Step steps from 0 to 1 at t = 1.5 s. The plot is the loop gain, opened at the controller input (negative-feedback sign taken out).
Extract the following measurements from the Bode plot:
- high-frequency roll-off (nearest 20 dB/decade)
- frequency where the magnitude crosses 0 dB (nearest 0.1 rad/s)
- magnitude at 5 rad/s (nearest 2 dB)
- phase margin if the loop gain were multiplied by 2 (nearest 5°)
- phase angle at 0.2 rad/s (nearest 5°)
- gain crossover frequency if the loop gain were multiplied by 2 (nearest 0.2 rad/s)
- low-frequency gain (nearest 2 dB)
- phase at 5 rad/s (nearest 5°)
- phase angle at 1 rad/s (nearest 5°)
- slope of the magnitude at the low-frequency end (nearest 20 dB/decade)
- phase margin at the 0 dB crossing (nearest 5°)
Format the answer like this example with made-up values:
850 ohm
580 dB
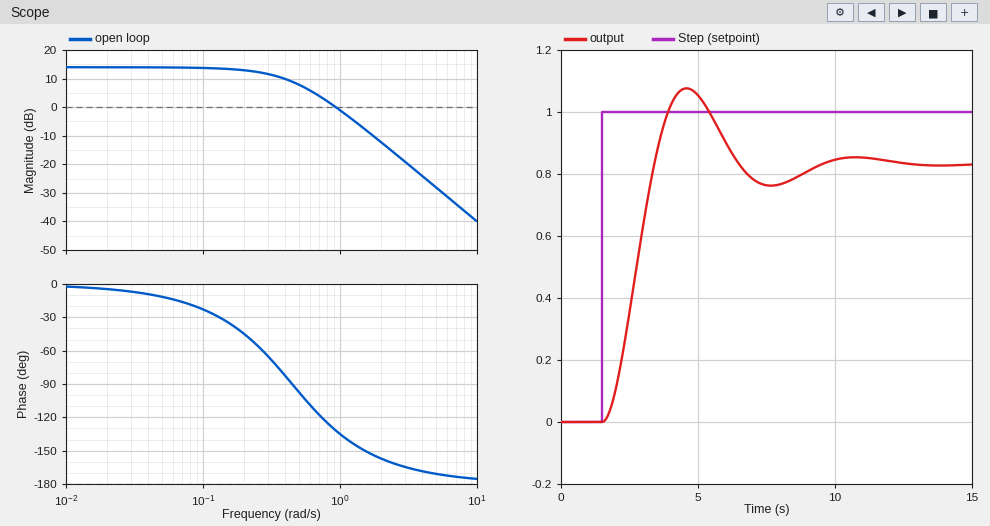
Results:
-40 dB/decade
0.9 rad/s
-28 dB
35°
-45°
1.4 rad/s
14 dB
-170°
-135°
0 dB/decade
50°
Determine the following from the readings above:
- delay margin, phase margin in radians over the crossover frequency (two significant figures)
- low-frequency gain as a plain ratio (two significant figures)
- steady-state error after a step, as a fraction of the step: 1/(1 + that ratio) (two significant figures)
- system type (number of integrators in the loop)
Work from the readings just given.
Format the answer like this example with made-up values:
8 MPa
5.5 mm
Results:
0.97 s
5.0
0.17
0
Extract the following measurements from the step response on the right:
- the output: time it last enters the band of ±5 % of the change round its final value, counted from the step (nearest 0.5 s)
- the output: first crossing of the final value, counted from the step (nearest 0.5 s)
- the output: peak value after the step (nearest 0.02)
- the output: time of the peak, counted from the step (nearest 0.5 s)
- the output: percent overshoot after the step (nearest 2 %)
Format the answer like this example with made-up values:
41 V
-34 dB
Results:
7.0 s
2.0 s
1.08
3.0 s
30 %
